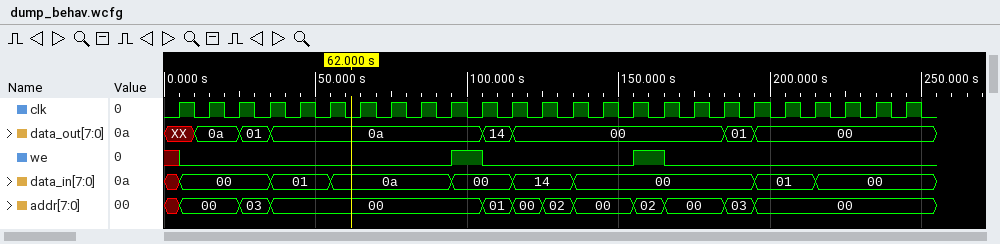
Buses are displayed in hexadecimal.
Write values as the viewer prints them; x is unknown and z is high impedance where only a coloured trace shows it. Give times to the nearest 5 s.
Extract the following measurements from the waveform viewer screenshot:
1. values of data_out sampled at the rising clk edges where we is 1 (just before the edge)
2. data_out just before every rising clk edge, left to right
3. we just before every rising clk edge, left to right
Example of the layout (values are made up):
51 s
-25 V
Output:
0a, 00
XX, 0a, 0a, 01, 0a, 0a, 0a, 0a, 0a, 0a, 0a, 14, 00, 00, 00, 00, 00, 00, 00, 01, 00, 00, 00, 00, 00
x 0 0 0 0 0 0 0 0 0 1 0 0 0 0 0 1 0 0 0 0 0 0 0 0
